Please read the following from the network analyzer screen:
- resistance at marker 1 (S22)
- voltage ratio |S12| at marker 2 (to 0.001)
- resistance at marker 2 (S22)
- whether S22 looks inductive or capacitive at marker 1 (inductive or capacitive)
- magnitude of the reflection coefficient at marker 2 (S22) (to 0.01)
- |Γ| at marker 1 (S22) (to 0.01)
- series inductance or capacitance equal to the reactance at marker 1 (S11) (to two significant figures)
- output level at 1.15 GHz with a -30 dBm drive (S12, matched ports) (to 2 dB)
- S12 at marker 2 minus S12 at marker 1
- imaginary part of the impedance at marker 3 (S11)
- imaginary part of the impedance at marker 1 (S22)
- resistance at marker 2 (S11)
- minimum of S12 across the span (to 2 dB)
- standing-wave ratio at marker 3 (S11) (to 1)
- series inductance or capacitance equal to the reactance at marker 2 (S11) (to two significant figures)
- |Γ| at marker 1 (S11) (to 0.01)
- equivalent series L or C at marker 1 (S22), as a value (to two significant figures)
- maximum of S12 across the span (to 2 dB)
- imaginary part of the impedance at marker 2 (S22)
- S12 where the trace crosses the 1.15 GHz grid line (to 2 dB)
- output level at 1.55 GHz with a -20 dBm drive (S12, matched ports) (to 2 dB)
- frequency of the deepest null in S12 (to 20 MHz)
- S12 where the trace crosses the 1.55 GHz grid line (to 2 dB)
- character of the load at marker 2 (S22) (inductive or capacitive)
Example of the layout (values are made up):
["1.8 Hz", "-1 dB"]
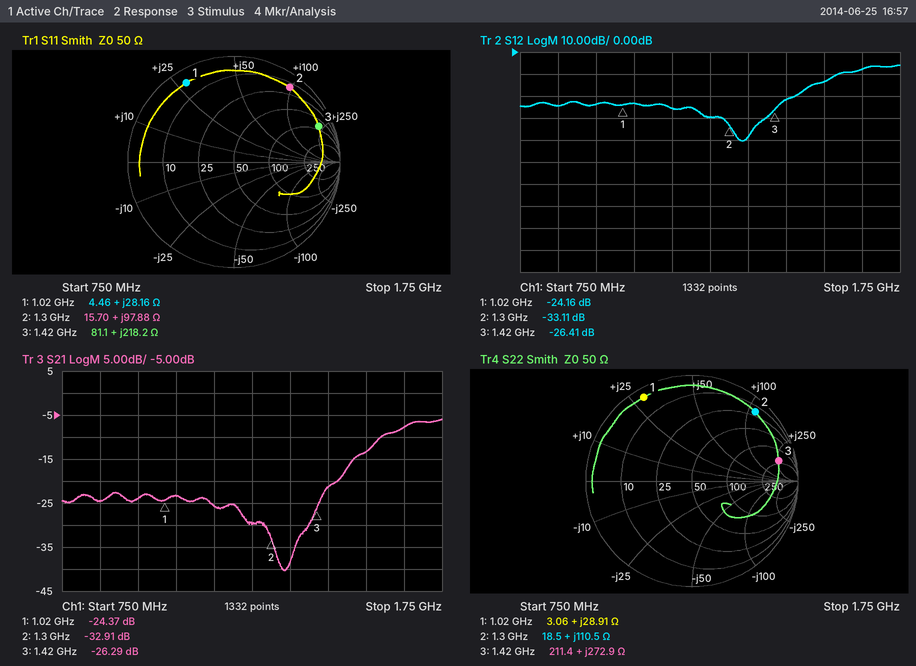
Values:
["3.06 Ω", "0.022", "18.5 Ω", "inductive", "0.88", "0.91", "4.4 nH", "-56 dBm", "-8.95 dB", "+218.2 Ω", "+28.91 Ω", "15.70 Ω", "-40 dB", "14", "12 nH", "0.87", "4.5 nH", "-6 dB", "+110.5 Ω", "-26 dB", "-34 dBm", "1.34 GHz", "-14 dB", "inductive"]
